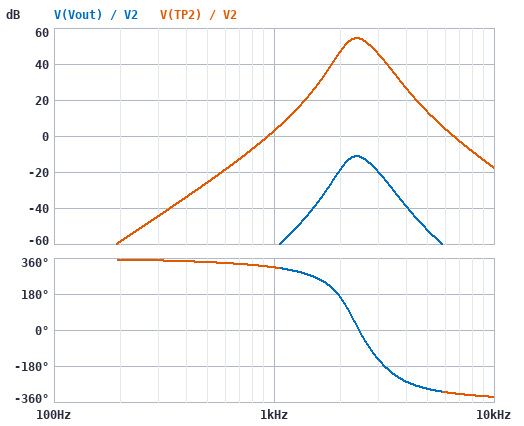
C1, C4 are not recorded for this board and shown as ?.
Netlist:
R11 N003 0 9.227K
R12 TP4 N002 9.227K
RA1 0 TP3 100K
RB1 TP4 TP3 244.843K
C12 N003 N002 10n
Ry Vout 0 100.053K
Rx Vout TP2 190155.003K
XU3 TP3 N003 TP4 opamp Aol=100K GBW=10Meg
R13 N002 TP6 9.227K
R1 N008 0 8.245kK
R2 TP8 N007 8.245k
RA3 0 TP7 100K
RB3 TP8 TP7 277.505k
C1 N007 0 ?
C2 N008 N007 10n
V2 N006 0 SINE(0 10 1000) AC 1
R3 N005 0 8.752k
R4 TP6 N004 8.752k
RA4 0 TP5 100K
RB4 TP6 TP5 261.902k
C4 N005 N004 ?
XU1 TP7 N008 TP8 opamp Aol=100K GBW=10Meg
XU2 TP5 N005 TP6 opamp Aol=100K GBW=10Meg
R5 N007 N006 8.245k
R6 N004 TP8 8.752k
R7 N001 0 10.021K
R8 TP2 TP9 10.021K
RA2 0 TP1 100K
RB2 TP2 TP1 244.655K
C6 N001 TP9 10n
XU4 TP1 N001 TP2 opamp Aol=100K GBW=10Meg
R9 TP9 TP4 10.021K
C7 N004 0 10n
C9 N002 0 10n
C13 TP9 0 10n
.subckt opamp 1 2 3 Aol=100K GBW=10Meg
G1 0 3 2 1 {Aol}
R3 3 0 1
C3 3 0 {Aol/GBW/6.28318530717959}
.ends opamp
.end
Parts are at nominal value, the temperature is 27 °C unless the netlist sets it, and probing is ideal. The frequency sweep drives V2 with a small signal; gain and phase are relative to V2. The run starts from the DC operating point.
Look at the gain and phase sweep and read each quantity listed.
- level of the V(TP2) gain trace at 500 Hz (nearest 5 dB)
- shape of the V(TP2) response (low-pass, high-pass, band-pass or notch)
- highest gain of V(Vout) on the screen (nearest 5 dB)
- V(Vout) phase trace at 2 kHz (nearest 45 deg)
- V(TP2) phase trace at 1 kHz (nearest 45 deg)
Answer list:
-25 dB
band-pass
-10 dB
180 deg
315 deg
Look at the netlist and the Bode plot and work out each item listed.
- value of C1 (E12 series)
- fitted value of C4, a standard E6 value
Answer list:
15 nF
6.8 nF
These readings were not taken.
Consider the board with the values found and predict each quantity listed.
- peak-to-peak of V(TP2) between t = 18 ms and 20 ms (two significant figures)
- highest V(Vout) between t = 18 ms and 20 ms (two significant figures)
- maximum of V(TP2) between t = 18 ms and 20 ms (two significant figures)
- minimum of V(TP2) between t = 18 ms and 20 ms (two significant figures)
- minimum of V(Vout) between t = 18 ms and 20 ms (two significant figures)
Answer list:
28 V
7.3 mV
14 V
-14 V
-7.3 mV
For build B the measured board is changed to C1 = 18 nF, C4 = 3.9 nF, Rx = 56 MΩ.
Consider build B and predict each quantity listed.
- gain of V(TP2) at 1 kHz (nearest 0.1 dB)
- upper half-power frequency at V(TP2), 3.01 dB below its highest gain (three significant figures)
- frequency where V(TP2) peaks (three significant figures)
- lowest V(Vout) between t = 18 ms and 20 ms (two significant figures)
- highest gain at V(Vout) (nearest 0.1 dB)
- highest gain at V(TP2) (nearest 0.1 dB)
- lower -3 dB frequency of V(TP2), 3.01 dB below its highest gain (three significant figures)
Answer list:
-2.3 dB
2.63 kHz
2.33 kHz
-14 mV
-12.5 dB
42.4 dB
2.07 kHz
